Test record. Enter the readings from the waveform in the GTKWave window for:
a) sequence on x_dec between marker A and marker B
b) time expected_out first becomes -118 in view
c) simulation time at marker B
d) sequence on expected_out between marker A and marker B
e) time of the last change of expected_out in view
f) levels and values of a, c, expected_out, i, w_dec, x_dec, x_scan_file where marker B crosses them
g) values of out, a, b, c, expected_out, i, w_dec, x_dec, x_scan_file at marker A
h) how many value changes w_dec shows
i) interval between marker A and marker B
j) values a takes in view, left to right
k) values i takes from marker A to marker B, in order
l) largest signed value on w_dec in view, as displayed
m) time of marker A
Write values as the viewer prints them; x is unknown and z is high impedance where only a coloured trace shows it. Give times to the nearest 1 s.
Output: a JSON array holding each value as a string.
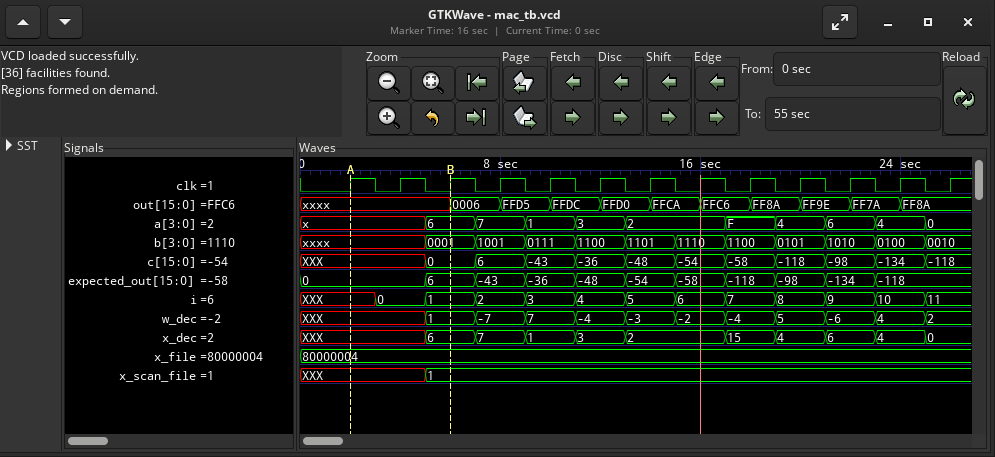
["XXX, 6", "17 s", "6 s", "0, 6", "23 s", "a=6, c=0, expected_out=6, i=1, w_dec=1, x_dec=6, x_scan_file=1", "out=xxxx, a=x, b=xxxx, c=XXX, expected_out=0, i=XXX, w_dec=XXX, x_dec=XXX, x_scan_file=XXX", "11", "4 s", "x, 6, 7, 1, 3, 2, F, 4, 6, 4, 0", "XXX, 0, 1", "7", "2 s"]
